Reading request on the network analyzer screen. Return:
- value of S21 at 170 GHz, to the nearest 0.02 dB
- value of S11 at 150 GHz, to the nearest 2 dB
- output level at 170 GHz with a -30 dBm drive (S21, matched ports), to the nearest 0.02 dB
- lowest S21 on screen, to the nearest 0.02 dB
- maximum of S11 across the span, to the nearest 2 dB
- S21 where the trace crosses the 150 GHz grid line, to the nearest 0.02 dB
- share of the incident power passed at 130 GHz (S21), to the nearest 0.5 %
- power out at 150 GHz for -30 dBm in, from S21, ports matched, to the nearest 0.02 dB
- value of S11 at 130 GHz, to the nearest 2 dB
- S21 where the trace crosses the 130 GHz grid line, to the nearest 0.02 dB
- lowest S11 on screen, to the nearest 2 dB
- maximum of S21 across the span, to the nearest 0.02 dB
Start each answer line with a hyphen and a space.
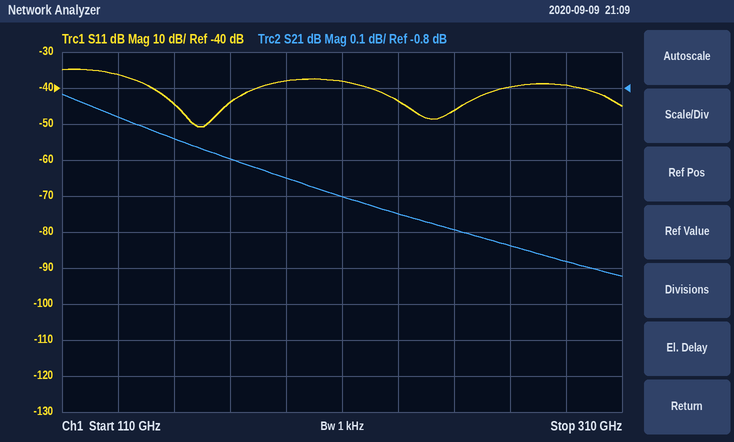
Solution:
- -1.00 dB
- -44 dB
- -31.00 dBm
- -1.32 dB
- -34 dB
- -0.94 dB
- 81.5 %
- -30.94 dBm
- -36 dB
- -0.88 dB
- -50 dB
- -0.82 dB
